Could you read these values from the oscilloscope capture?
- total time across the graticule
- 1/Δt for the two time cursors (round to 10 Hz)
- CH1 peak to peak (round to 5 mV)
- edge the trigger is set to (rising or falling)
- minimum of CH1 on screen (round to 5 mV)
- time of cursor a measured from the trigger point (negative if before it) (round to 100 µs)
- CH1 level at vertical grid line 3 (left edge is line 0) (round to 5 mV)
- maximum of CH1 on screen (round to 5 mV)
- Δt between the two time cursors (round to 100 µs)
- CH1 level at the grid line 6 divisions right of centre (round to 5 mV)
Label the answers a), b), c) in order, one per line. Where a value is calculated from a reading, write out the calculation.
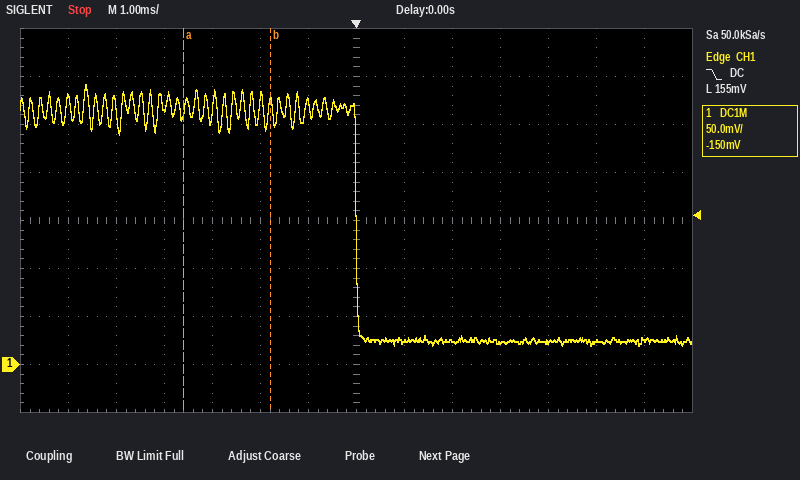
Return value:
a) 14 ms
b) 1 / 1.8 ms ≈ 560 Hz
c) 290 mV − (20 mV) = 270 mV
d) falling
e) 20 mV
f) -3.6 ms
g) 270 mV
h) 290 mV
i) 1.8 ms
j) 25 mV
